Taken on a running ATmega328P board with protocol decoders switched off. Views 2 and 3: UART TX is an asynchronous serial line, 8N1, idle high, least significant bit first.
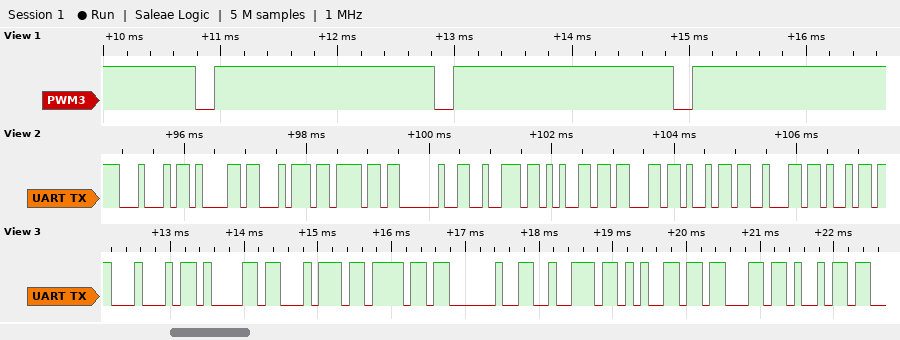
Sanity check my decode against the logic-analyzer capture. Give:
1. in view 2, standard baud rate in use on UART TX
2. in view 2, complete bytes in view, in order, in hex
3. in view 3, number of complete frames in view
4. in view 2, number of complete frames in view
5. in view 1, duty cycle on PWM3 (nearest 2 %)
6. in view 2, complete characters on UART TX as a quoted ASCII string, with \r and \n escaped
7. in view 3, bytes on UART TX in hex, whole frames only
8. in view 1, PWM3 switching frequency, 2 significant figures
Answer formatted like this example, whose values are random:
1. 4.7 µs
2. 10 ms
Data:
1. 9600 baud
2. 0x44 0x61 0x74 0x6F 0x20 0x72 0x65 0x63 0x69 0x62 0x69
3. 9
4. 11
5. 92 %
6. "Dato recibi"
7. 44 61 74 6F 20 72 65 63 69
8. 490 Hz
